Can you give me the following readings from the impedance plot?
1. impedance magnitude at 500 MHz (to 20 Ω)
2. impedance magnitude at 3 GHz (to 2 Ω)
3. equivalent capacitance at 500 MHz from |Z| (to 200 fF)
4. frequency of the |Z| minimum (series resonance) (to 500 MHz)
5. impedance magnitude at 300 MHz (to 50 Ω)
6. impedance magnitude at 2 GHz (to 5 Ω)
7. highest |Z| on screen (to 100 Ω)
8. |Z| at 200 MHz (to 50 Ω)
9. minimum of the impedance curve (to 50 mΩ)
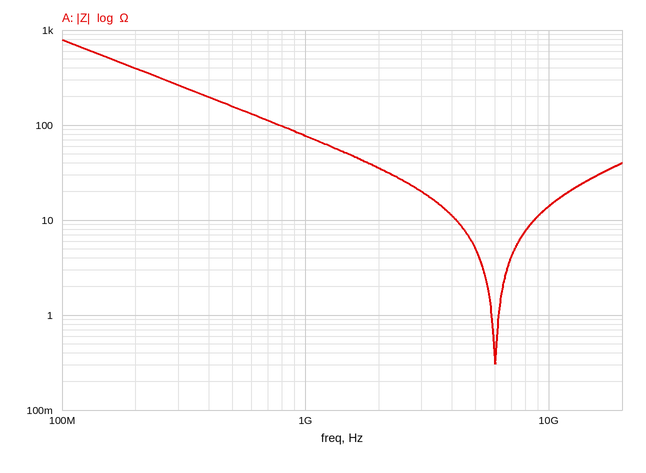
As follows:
160 Ω
20 Ω
2.0 pF
6.0 GHz
250 Ω
35 Ω
800 Ω
400 Ω
300 mΩ
